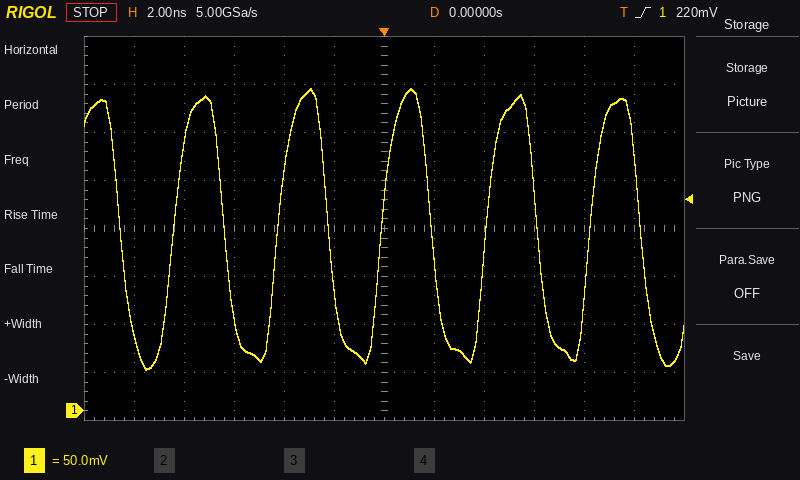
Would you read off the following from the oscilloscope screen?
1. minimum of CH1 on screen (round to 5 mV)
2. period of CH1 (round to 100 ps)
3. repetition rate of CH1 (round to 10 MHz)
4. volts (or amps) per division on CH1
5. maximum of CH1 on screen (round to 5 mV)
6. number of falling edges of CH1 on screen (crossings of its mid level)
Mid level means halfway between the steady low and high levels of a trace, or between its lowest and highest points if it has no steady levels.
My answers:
45 mV
4.2 ns
240 MHz
50 mV
335 mV
6
